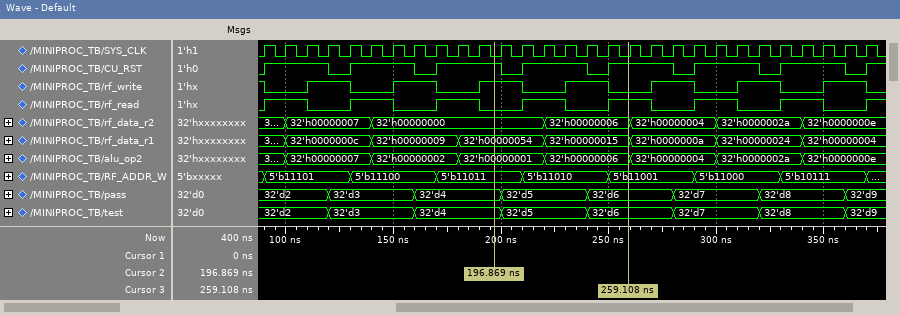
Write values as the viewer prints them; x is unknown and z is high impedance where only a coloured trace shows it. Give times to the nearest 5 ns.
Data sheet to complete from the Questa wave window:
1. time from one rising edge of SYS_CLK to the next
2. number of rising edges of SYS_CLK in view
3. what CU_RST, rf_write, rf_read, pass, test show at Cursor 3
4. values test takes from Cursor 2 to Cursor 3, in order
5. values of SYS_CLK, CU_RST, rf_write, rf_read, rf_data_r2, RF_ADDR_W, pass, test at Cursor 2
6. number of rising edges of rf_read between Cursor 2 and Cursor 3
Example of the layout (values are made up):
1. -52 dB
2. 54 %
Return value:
1. 10 ns
2. 29
3. CU_RST=1, rf_write=0, rf_read=1, pass=32'd6, test=32'd6
4. 32'd4, 32'd5, 32'd6
5. SYS_CLK=0, CU_RST=1, rf_write=1, rf_read=0, rf_data_r2=32'h00000000, RF_ADDR_W=5'b11011, pass=32'd4, test=32'd4
6. 2
